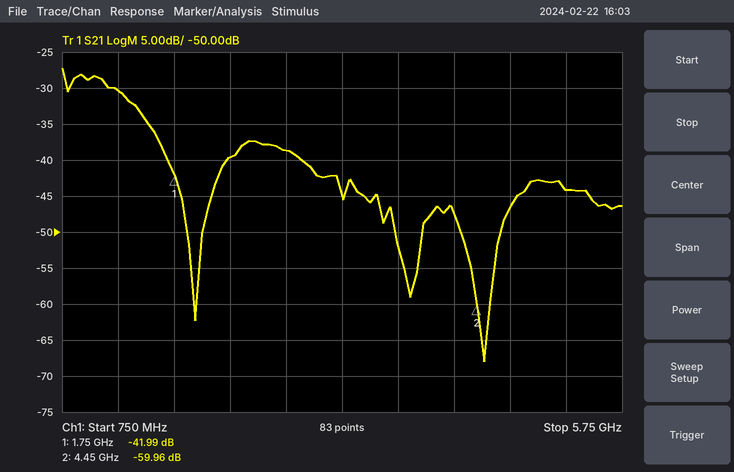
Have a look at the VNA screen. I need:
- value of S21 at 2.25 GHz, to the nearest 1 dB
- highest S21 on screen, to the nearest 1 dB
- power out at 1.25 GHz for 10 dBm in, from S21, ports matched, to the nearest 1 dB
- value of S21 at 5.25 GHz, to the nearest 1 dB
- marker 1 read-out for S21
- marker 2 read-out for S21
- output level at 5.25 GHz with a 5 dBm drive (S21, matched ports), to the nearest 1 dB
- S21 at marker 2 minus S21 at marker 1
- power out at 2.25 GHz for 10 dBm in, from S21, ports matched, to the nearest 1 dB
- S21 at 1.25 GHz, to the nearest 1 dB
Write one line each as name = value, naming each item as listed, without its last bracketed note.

value of S21 at 2.25 GHz, to the nearest 1 dB = -40 dB
highest S21 on screen, to the nearest 1 dB = -27 dB
power out at 1.25 GHz for 10 dBm in, from S21, ports matched, to the nearest 1 dB = -20 dBm
value of S21 at 5.25 GHz, to the nearest 1 dB = -44 dB
marker 1 read-out for S21 = -41.99 dB
marker 2 read-out for S21 = -59.96 dB
output level at 5.25 GHz with a 5 dBm drive (S21, matched ports), to the nearest 1 dB = -39 dBm
S21 at marker 2 minus S21 at marker 1 = -17.97 dB
power out at 2.25 GHz for 10 dBm in, from S21, ports matched, to the nearest 1 dB = -30 dBm
S21 at 1.25 GHz, to the nearest 1 dB = -30 dB
